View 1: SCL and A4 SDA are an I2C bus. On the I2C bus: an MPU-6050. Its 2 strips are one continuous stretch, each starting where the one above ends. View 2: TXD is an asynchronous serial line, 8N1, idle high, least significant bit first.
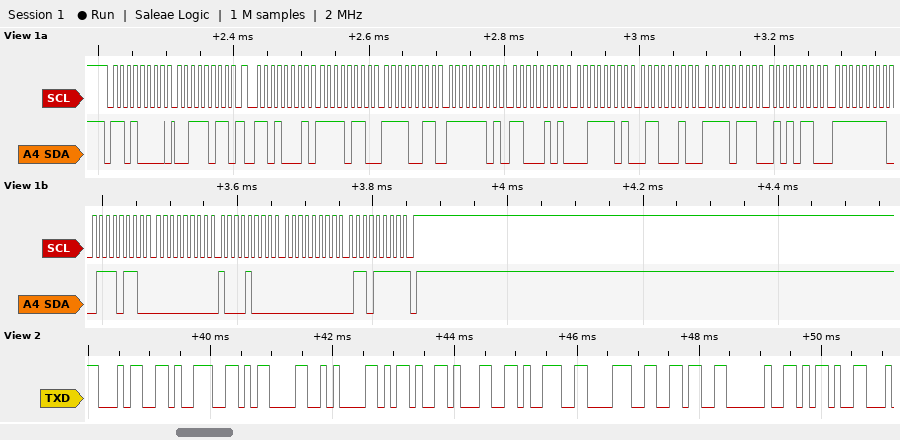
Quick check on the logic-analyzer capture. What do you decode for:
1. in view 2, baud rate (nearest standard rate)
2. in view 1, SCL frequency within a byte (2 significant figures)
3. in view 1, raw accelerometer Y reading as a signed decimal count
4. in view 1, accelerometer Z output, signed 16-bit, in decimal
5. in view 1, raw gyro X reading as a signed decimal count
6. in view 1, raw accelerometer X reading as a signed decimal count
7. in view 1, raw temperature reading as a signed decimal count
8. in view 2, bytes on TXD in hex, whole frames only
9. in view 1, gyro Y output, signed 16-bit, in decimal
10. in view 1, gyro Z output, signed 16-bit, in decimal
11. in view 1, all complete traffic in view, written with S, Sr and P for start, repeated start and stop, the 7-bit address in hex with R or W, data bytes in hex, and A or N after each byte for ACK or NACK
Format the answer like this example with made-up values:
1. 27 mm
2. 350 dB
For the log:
1. 9600 baud
2. 100 kHz
3. -571
4. 15714
5. -138
6. -2317
7. -2218
8. 0x34 0x39 0x0D 0x0A 0x2D 0x31 0x39 0x38 0x36 0x20 0x2D
9. 136
10. 111
11. S 68W A 3B A Sr 68R A F6 A F3 A FD A C5 A 3D A 62 A F7 A 56 A FF A 76 A 00 A 88 A 00 A 6F N P
